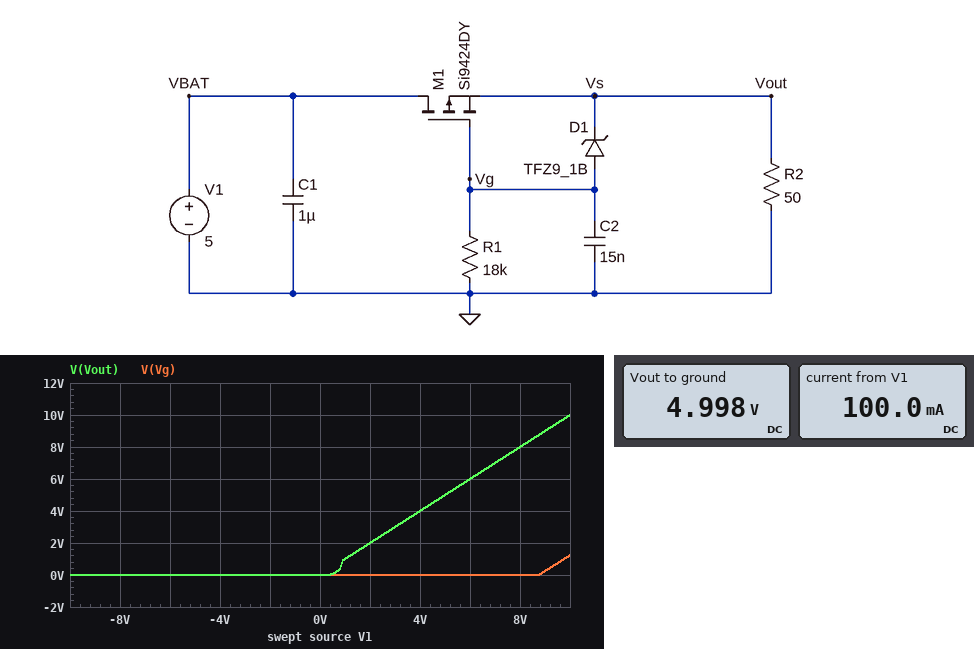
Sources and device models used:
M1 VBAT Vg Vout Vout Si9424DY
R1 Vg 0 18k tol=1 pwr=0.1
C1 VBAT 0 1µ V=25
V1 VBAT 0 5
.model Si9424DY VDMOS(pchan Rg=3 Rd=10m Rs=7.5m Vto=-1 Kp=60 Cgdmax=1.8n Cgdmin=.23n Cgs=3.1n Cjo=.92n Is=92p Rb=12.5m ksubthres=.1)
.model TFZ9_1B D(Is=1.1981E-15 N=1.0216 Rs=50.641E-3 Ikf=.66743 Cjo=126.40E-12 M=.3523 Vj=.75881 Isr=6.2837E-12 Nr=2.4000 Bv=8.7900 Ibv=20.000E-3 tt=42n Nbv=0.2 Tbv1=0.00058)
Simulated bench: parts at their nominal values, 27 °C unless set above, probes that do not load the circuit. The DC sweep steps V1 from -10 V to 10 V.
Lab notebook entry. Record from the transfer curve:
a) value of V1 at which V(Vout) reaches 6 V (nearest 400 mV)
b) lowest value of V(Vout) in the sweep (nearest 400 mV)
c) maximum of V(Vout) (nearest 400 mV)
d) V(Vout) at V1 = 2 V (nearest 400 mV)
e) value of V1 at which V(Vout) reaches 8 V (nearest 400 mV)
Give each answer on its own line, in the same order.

6.0 V
0 V
10.0 V
2.0 V
8.0 V
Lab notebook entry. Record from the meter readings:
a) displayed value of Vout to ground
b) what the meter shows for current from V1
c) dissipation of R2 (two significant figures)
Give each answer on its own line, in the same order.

4.998 V
100.0 mA
500 mW
